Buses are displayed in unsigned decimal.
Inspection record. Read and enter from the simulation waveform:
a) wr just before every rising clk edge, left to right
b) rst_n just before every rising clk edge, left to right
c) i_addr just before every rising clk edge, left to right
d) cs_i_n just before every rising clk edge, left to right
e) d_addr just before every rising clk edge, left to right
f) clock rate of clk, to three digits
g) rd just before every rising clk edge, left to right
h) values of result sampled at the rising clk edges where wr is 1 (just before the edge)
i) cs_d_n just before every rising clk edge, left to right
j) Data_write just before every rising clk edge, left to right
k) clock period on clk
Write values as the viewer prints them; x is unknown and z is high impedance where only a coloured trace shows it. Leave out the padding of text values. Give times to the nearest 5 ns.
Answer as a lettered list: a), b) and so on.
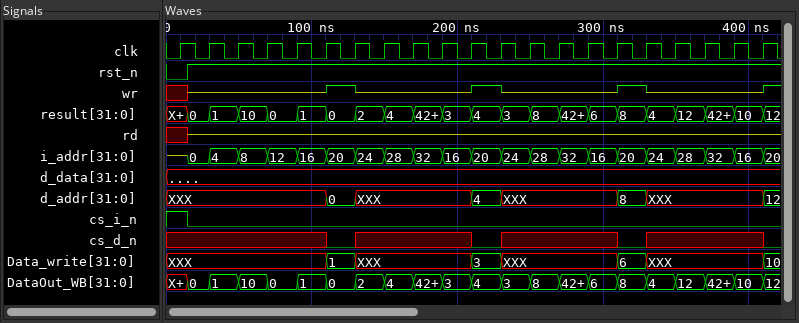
a) x z z z z z 1 z z z z 1 z z z z 1 z z z z
b) 0 1 1 1 1 1 1 1 1 1 1 1 1 1 1 1 1 1 1 1 1
c) z, 0, 4, 8, 12, 16, 20, 24, 28, 32, 16, 20, 24, 28, 32, 16, 20, 24, 28, 32, 16
d) 1 0 0 0 0 0 0 0 0 0 0 0 0 0 0 0 0 0 0 0 0
e) XXX, XXX, XXX, XXX, XXX, XXX, 0, XXX, XXX, XXX, XXX, 4, XXX, XXX, XXX, XXX, 8, XXX, XXX, XXX, XXX
f) 50.0 MHz
g) x z z z z z z z z z z z z z z z z z z z z
h) 0, 4, 8
i) x x x x x x 0 x x x x 0 x x x x 0 x x x x
j) XXX, XXX, XXX, XXX, XXX, XXX, 1, XXX, XXX, XXX, XXX, 3, XXX, XXX, XXX, XXX, 6, XXX, XXX, XXX, XXX
k) 20 ns
